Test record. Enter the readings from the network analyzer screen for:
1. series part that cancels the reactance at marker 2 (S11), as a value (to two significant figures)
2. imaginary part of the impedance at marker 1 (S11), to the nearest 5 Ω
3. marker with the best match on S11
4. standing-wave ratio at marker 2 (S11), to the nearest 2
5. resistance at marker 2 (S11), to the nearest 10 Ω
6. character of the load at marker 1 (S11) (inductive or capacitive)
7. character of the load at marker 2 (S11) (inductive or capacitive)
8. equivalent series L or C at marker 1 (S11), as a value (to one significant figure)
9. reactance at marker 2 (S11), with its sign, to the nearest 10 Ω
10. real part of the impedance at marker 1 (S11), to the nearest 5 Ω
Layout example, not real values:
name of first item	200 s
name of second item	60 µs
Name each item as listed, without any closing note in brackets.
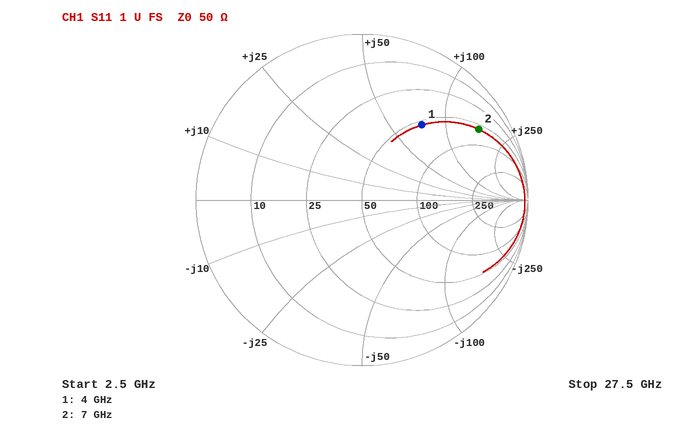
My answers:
series part that cancels the reactance at marker 2 (S11), as a value	140 fF
imaginary part of the impedance at marker 1 (S11), to the nearest 5 Ω	+75 Ω
marker with the best match on S11	marker 1
standing-wave ratio at marker 2 (S11), to the nearest 2	10
resistance at marker 2 (S11), to the nearest 10 Ω	60 Ω
character of the load at marker 1 (S11)	inductive
character of the load at marker 2 (S11)	inductive
equivalent series L or C at marker 1 (S11), as a value	3 nH
reactance at marker 2 (S11), with its sign, to the nearest 10 Ω	+160 Ω
real part of the impedance at marker 1 (S11), to the nearest 5 Ω	55 Ω
